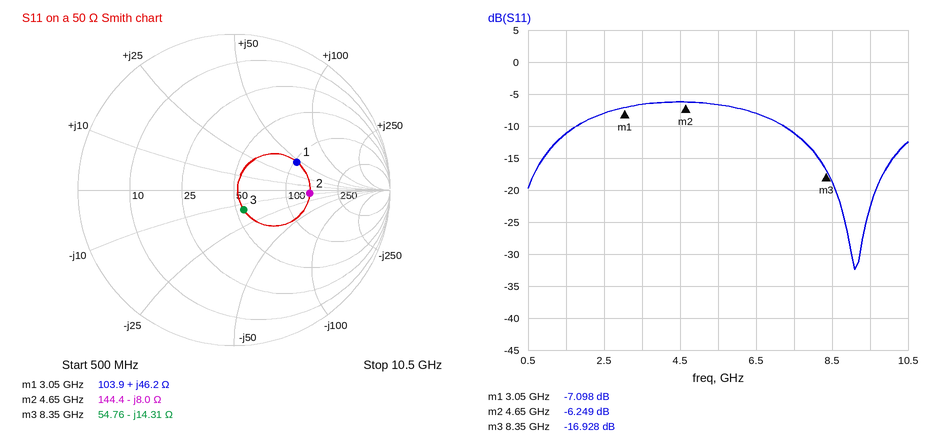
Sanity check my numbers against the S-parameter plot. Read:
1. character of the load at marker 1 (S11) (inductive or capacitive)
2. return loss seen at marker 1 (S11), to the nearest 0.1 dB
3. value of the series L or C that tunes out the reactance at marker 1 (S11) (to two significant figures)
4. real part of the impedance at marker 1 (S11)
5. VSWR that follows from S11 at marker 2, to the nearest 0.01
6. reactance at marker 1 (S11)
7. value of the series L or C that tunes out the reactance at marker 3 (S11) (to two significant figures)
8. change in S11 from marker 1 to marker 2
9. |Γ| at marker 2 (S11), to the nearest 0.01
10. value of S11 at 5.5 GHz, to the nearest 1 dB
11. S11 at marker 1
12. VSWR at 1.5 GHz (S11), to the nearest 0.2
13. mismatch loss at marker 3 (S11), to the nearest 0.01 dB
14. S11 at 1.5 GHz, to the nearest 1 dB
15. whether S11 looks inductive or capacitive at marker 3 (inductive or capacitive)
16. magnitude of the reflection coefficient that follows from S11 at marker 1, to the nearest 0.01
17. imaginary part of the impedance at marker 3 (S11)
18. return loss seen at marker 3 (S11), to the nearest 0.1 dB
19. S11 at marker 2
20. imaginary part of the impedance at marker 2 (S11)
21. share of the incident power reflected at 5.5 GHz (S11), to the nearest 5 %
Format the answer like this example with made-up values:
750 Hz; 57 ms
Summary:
inductive; 7.1 dB; 1.1 pF; 103.9 Ω; 2.90; +46.2 Ω; 270 pH; 0.849 dB; 0.49; -7 dB; -7.098 dB; 1.8; 0.09 dB; -11 dB; capacitive; 0.44; -14.31 Ω; 16.9 dB; -6.249 dB; -8.0 Ω; 20 %
